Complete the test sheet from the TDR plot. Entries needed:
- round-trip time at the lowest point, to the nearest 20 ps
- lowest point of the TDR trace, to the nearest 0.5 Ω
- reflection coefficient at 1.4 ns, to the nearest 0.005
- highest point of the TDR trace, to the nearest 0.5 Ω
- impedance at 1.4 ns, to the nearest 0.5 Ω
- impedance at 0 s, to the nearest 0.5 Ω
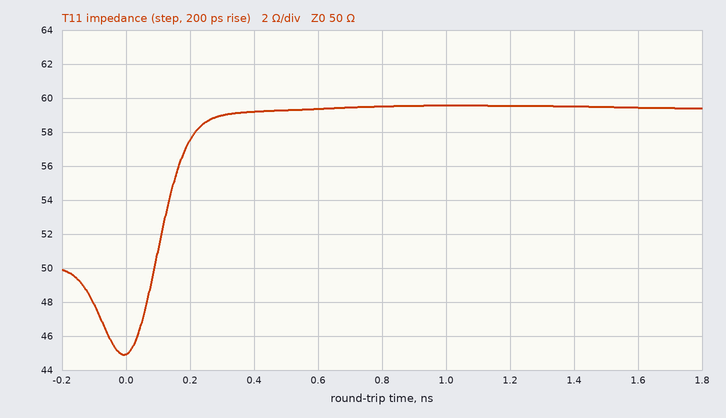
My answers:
0 ps
45.0 Ω
+0.085
59.5 Ω
59.5 Ω
45.0 Ω
